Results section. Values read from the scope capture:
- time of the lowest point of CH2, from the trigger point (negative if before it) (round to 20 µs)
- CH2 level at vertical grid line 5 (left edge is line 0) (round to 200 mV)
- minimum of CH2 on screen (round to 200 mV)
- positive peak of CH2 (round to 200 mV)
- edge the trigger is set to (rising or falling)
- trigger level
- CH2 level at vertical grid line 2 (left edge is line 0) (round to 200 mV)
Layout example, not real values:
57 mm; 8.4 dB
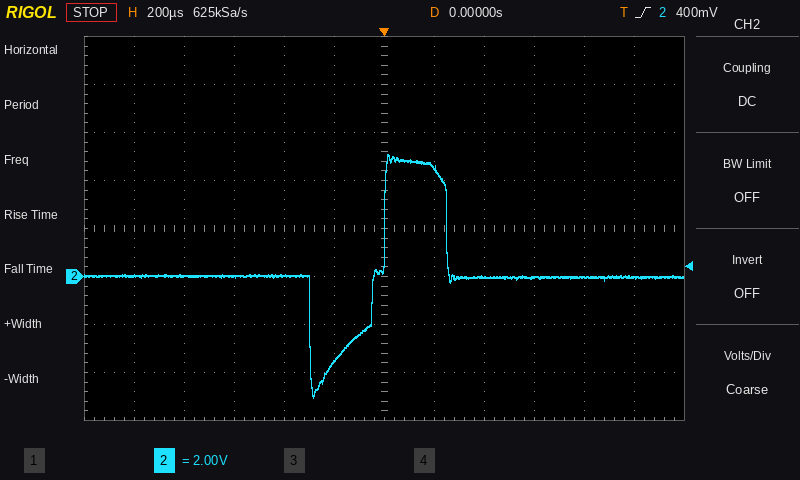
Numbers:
-280 µs; -3.6 V; -5.0 V; 5.0 V; rising; 400 mV; 0.0 V
